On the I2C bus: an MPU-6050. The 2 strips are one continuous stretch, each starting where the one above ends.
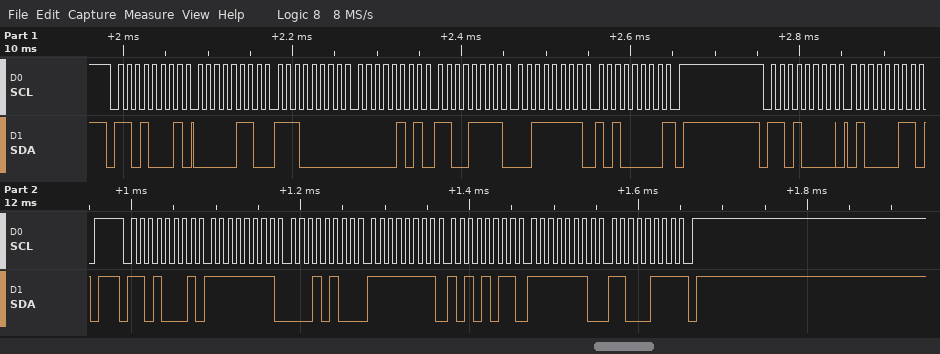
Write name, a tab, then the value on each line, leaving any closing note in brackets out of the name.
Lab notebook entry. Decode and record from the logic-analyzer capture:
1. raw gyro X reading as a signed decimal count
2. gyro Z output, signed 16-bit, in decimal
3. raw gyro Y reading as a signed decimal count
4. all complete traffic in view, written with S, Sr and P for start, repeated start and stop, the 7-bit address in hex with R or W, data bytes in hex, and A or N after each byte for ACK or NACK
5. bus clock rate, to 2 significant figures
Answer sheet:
raw gyro X reading as a signed decimal count	-236
gyro Z output, signed 16-bit, in decimal	-313
raw gyro Y reading as a signed decimal count	-85
all complete traffic in view, written with S, Sr and P for start, repeated start and stop, the 7-bit address in hex with R or W, data bytes in hex, and A or N after each byte for ACK or NACK	S 68R A 06 A E0 A 05 A CF A 3F A A0 N P S 68W A 43 A P S 68R A FF A 14 A FF A AB A FE A C7 N P
bus clock rate, to 2 significant figures	100 kHz
